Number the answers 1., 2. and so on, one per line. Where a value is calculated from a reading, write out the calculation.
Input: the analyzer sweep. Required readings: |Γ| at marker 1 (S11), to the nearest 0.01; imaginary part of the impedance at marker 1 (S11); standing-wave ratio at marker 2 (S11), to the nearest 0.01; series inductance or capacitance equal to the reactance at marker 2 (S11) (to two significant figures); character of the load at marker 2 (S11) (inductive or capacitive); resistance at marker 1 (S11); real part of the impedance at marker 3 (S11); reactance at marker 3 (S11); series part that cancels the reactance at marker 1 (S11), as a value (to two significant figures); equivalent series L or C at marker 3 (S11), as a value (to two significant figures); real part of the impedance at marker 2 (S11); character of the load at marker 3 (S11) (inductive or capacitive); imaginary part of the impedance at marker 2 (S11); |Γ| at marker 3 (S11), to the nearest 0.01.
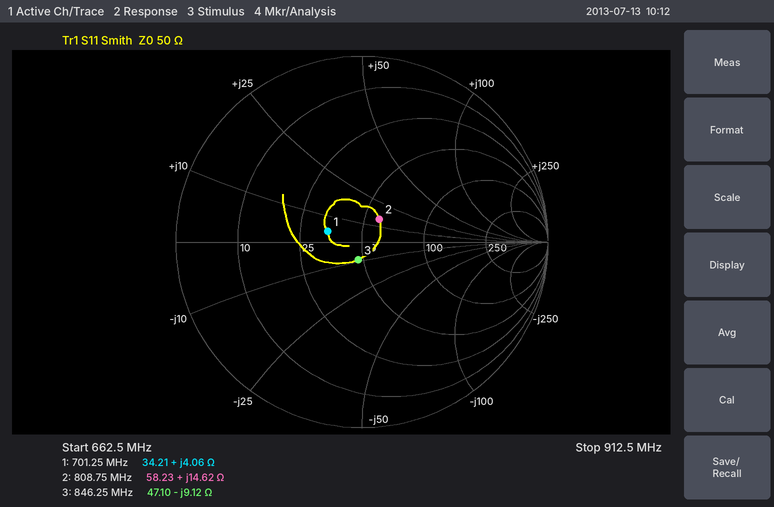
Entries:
1. 0.19
2. +4.06 Ω
3. 1.36
4. L = 14.62 Ω/(2π × 808.75 MHz) ≈ 2.9 nH
5. inductive
6. 34.21 Ω
7. 47.10 Ω
8. -9.12 Ω
9. C = 1/(2π × 701.25 MHz × 4.06 Ω) ≈ 56 pF
10. C = 1/(2π × 846.25 MHz × 9.12 Ω) ≈ 21 pF
11. 58.23 Ω
12. capacitive
13. +14.62 Ω
14. 0.10
